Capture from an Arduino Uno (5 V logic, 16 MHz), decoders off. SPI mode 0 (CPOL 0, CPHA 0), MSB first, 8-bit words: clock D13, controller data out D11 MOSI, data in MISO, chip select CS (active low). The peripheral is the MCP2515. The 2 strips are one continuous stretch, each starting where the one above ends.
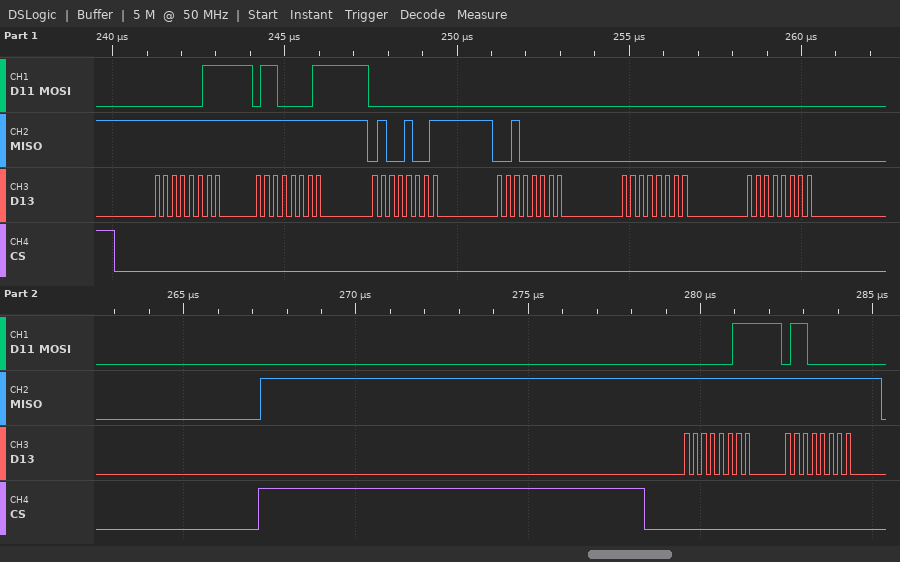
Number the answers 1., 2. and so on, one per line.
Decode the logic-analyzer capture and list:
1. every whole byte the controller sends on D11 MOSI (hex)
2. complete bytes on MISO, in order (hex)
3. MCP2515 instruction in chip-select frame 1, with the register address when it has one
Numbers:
1. 03 61 00 00 00 00 03 60
2. FF FF 49 20 00 00 FF FF
3. READ 0x61
